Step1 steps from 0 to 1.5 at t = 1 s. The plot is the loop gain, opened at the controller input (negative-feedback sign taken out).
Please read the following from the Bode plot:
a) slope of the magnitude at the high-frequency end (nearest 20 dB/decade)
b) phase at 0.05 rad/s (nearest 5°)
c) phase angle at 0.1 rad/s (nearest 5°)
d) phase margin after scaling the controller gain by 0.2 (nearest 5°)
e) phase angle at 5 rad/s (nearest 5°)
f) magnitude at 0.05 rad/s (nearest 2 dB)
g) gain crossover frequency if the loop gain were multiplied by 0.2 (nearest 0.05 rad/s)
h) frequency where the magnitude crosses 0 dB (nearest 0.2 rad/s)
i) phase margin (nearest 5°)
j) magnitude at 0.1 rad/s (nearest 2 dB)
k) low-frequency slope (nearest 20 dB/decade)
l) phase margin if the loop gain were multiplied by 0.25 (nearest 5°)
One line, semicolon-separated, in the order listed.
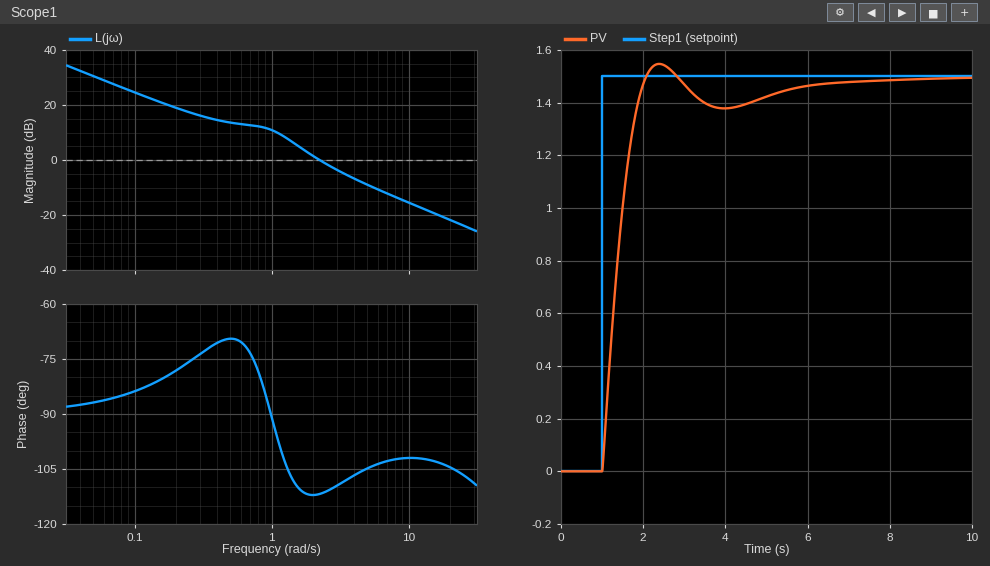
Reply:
-20 dB/decade; -85°; -85°; 110°; -105°; 30 dB; 0.45 rad/s; 2.2 rad/s; 70°; 24 dB; -20 dB/decade; 100°
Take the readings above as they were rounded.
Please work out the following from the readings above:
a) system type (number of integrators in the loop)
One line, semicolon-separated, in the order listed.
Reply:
1
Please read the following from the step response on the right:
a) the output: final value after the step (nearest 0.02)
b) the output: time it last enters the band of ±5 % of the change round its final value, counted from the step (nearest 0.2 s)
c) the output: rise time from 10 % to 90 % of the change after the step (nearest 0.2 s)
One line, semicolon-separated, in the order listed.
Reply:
1.50; 4.0 s; 0.8 s
